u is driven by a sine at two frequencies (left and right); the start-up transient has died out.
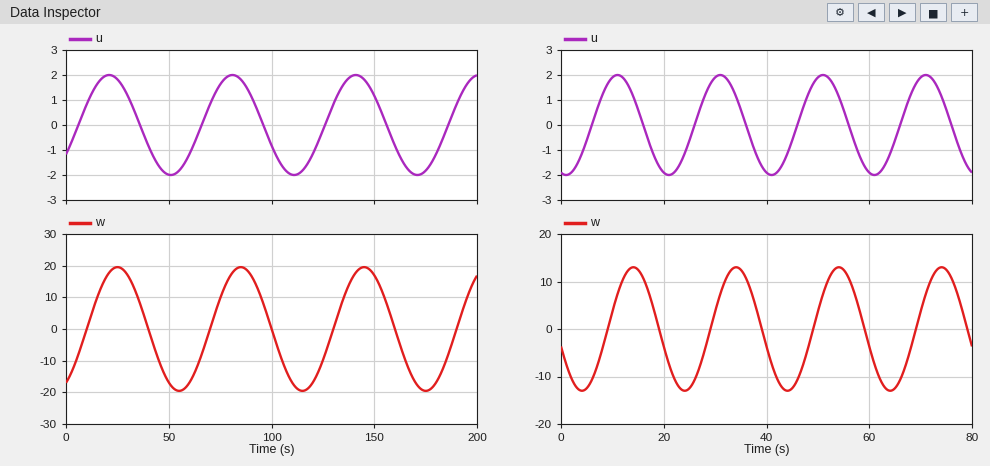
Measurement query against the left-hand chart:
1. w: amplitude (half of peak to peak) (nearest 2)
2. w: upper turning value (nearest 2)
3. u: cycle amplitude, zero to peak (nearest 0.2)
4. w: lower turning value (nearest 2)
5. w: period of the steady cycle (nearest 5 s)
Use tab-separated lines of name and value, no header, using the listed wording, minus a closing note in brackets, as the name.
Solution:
w: amplitude (half of peak to peak)	20
w: upper turning value	20
u: cycle amplitude, zero to peak	2.0
w: lower turning value	-20
w: period of the steady cycle	60 s
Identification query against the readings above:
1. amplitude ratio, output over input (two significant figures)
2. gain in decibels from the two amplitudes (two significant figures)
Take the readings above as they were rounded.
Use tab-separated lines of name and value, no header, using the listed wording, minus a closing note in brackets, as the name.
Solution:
amplitude ratio, output over input	10
gain in decibels from the two amplitudes	20 dB
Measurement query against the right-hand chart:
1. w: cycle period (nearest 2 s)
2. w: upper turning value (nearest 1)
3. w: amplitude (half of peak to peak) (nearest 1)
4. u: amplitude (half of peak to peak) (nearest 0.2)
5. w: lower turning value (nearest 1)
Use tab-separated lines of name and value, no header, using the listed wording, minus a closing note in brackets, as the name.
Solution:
w: cycle period	20 s
w: upper turning value	13
w: amplitude (half of peak to peak)	13
u: amplitude (half of peak to peak)	2.0
w: lower turning value	-13
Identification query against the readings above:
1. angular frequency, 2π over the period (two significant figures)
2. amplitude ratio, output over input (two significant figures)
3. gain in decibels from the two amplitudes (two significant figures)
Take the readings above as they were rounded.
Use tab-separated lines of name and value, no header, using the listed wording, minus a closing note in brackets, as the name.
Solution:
angular frequency, 2π over the period	0.31 rad/s
amplitude ratio, output over input	6.5
gain in decibels from the two amplitudes	16 dB
